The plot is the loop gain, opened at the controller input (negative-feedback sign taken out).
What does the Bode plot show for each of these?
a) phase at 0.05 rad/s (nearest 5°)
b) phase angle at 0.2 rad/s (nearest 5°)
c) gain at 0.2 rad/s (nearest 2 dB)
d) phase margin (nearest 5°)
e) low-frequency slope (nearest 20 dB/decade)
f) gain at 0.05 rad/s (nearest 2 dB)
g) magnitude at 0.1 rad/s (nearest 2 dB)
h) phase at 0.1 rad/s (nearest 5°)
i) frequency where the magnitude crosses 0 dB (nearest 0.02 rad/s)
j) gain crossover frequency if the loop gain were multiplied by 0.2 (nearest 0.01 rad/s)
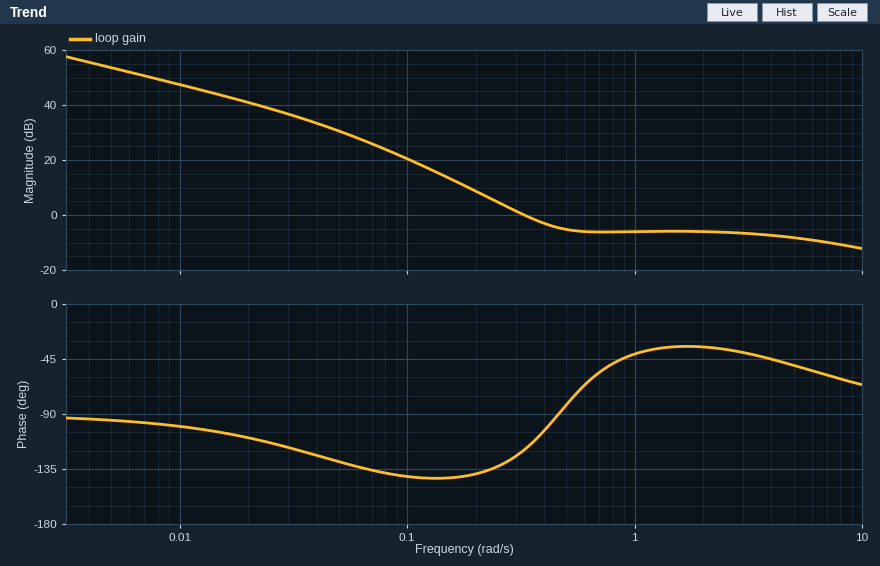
-130°
-140°
8 dB
60°
-20 dB/decade
30 dB
20 dB
-140°
0.32 rad/s
0.15 rad/s
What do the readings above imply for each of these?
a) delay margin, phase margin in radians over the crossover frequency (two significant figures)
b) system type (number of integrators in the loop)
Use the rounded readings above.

3.3 s
1
